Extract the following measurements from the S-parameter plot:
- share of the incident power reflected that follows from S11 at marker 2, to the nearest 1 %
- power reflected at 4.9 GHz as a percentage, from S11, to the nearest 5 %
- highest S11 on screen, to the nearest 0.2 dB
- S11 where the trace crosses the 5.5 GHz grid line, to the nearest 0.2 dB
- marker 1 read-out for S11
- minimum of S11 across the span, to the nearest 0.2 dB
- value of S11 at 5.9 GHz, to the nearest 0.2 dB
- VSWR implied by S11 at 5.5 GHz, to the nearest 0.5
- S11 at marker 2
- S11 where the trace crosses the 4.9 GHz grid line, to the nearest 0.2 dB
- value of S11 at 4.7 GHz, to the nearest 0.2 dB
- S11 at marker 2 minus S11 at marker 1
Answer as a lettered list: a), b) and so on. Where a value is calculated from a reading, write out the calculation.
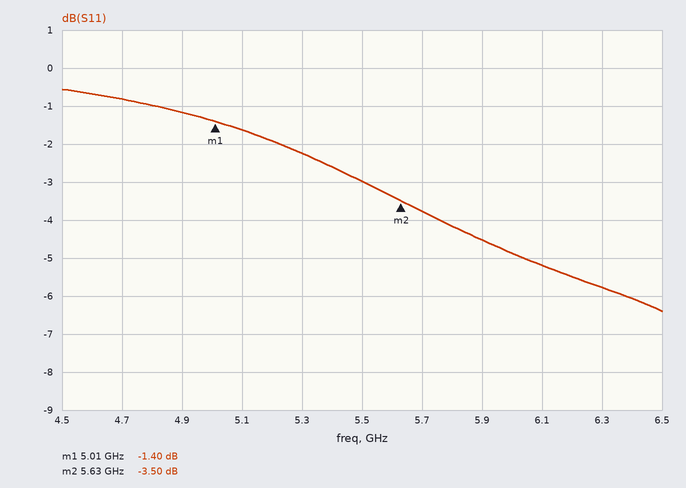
a) 10^(-3.5/10) ≈ 45 %
b) 10^(-1.2/10) ≈ 75.9 %, so 75 % to the nearest 5 %
c) -0.6 dB
d) -3.0 dB
e) -1.40 dB
f) -6.4 dB
g) -4.6 dB
h) |Γ| = 10^(-3/20) = 0.7079; VSWR = (1 + 0.7079)/(1 − 0.7079) ≈ 5.85, so 6.0 to the nearest 0.5
i) -3.50 dB
j) -1.2 dB
k) -0.8 dB
l) -3.5 − (-1.4) = -2.10 dB
